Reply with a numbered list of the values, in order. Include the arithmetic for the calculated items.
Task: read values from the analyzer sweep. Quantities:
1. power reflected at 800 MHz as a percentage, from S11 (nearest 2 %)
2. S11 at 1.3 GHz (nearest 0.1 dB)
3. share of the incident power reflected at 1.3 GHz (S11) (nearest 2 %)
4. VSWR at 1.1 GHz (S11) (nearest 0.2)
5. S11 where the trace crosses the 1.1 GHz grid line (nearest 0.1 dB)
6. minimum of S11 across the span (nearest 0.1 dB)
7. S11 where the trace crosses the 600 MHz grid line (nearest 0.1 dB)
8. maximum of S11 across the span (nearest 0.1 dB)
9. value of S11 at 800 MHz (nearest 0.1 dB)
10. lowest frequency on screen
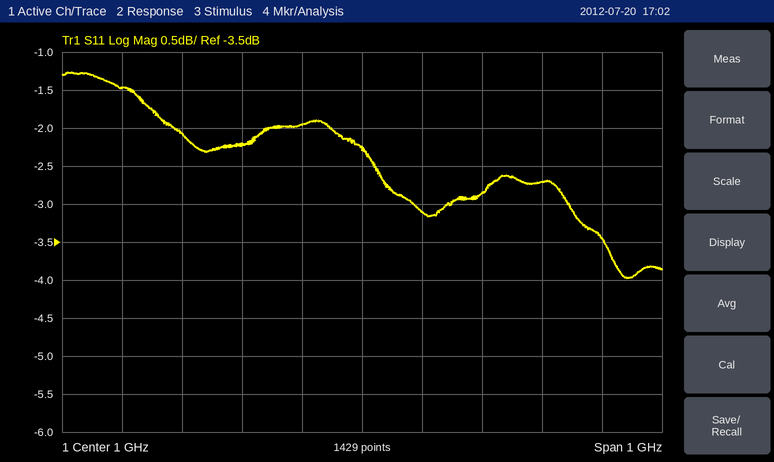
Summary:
1. 10^(-2.2/10) ≈ 60 %
2. -2.7 dB
3. 10^(-2.7/10) ≈ 54 %
4. |Γ| = 10^(-3.1/20) = 0.6998; VSWR = (1 + 0.6998)/(1 − 0.6998) ≈ 5.66, so 5.6 to the nearest 0.2
5. -3.1 dB
6. -4.0 dB
7. -1.5 dB
8. -1.3 dB
9. -2.2 dB
10. 500 MHz
